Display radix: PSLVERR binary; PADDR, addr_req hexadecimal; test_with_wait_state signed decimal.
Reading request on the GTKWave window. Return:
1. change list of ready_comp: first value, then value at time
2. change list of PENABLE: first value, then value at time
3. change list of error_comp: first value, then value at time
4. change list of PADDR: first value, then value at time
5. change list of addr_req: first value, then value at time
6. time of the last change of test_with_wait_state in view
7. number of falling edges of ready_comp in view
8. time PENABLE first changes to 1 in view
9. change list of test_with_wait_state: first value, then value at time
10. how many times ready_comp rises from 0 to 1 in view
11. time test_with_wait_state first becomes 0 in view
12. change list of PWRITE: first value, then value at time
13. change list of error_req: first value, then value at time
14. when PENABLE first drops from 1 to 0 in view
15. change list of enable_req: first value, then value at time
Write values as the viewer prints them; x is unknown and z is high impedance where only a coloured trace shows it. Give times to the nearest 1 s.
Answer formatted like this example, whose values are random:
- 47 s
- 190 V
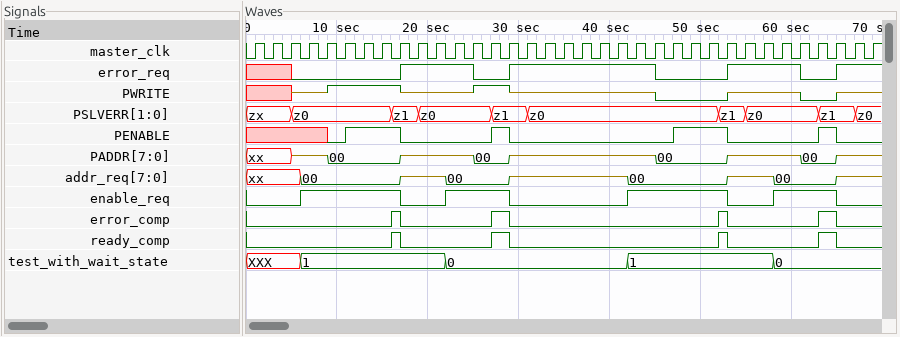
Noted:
- 0, 1 at 16 s, 0 at 17 s, 1 at 27 s, 0 at 29 s, 1 at 52 s, 0 at 53 s, 1 at 63 s, 0 at 65 s
- x, 0 at 9 s, 1 at 11 s, 0 at 17 s, 1 at 27 s, 0 at 29 s, 1 at 47 s, 0 at 53 s, 1 at 63 s, 0 at 65 s
- 0, 1 at 16 s, 0 at 17 s, 1 at 27 s, 0 at 29 s, 1 at 52 s, 0 at 53 s, 1 at 63 s, 0 at 65 s
- xx, z at 5 s, 00 at 9 s, z at 17 s, 00 at 25 s, z at 29 s, 00 at 45 s, z at 53 s, 00 at 61 s, z at 65 s
- xx, 00 at 6 s, z at 17 s, 00 at 22 s, z at 29 s, 00 at 42 s, z at 53 s, 00 at 58 s, z at 65 s
- 58 s
- 4
- 11 s
- XXX, 1 at 6 s, 0 at 22 s, 1 at 42 s, 0 at 58 s
- 4
- 22 s
- x, z at 5 s, 1 at 9 s, z at 17 s, 1 at 25 s, z at 29 s, 0 at 45 s, z at 53 s, 0 at 61 s, z at 65 s
- x, 0 at 5 s, 1 at 17 s, 0 at 25 s, 1 at 29 s, 0 at 45 s, 1 at 53 s, 0 at 61 s, 1 at 65 s
- 17 s
- 0, 1 at 6 s, 0 at 17 s, 1 at 22 s, 0 at 29 s, 1 at 42 s, 0 at 53 s, 1 at 58 s, 0 at 65 s
